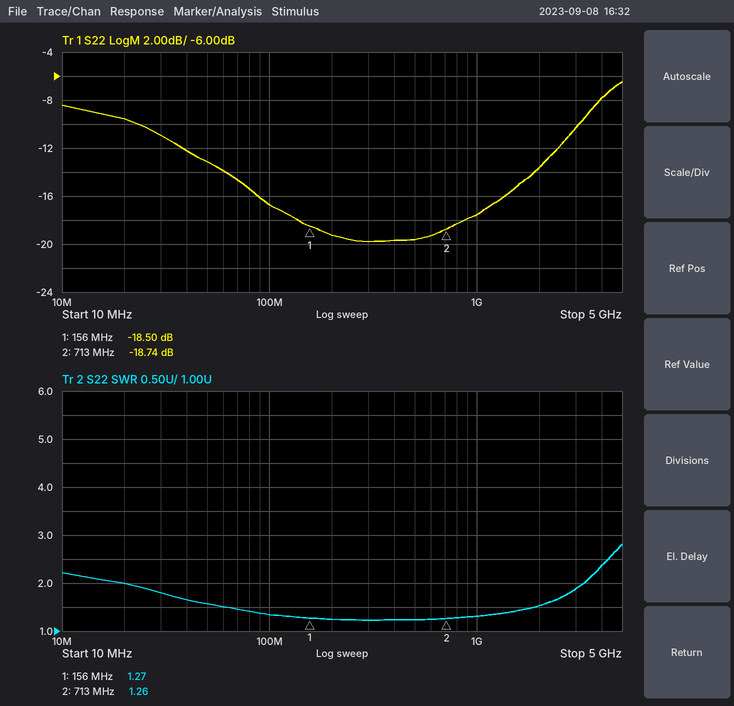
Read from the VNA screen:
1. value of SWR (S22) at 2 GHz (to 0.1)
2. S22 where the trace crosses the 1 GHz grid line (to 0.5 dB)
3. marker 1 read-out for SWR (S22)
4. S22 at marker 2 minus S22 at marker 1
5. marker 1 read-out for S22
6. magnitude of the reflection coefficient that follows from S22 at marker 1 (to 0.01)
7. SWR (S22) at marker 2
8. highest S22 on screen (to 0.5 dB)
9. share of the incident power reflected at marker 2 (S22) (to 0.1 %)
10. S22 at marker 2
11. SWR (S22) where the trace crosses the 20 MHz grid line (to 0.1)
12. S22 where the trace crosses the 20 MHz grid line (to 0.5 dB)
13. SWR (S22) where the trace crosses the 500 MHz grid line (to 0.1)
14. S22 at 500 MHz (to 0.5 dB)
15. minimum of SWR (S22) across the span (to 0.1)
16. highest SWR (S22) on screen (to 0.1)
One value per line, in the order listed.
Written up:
1.5
-17.5 dB
1.27
-0.24 dB
-18.50 dB
0.12
1.26
-6.5 dB
1.3 %
-18.74 dB
2.0
-9.5 dB
1.2
-19.5 dB
1.2
2.8
